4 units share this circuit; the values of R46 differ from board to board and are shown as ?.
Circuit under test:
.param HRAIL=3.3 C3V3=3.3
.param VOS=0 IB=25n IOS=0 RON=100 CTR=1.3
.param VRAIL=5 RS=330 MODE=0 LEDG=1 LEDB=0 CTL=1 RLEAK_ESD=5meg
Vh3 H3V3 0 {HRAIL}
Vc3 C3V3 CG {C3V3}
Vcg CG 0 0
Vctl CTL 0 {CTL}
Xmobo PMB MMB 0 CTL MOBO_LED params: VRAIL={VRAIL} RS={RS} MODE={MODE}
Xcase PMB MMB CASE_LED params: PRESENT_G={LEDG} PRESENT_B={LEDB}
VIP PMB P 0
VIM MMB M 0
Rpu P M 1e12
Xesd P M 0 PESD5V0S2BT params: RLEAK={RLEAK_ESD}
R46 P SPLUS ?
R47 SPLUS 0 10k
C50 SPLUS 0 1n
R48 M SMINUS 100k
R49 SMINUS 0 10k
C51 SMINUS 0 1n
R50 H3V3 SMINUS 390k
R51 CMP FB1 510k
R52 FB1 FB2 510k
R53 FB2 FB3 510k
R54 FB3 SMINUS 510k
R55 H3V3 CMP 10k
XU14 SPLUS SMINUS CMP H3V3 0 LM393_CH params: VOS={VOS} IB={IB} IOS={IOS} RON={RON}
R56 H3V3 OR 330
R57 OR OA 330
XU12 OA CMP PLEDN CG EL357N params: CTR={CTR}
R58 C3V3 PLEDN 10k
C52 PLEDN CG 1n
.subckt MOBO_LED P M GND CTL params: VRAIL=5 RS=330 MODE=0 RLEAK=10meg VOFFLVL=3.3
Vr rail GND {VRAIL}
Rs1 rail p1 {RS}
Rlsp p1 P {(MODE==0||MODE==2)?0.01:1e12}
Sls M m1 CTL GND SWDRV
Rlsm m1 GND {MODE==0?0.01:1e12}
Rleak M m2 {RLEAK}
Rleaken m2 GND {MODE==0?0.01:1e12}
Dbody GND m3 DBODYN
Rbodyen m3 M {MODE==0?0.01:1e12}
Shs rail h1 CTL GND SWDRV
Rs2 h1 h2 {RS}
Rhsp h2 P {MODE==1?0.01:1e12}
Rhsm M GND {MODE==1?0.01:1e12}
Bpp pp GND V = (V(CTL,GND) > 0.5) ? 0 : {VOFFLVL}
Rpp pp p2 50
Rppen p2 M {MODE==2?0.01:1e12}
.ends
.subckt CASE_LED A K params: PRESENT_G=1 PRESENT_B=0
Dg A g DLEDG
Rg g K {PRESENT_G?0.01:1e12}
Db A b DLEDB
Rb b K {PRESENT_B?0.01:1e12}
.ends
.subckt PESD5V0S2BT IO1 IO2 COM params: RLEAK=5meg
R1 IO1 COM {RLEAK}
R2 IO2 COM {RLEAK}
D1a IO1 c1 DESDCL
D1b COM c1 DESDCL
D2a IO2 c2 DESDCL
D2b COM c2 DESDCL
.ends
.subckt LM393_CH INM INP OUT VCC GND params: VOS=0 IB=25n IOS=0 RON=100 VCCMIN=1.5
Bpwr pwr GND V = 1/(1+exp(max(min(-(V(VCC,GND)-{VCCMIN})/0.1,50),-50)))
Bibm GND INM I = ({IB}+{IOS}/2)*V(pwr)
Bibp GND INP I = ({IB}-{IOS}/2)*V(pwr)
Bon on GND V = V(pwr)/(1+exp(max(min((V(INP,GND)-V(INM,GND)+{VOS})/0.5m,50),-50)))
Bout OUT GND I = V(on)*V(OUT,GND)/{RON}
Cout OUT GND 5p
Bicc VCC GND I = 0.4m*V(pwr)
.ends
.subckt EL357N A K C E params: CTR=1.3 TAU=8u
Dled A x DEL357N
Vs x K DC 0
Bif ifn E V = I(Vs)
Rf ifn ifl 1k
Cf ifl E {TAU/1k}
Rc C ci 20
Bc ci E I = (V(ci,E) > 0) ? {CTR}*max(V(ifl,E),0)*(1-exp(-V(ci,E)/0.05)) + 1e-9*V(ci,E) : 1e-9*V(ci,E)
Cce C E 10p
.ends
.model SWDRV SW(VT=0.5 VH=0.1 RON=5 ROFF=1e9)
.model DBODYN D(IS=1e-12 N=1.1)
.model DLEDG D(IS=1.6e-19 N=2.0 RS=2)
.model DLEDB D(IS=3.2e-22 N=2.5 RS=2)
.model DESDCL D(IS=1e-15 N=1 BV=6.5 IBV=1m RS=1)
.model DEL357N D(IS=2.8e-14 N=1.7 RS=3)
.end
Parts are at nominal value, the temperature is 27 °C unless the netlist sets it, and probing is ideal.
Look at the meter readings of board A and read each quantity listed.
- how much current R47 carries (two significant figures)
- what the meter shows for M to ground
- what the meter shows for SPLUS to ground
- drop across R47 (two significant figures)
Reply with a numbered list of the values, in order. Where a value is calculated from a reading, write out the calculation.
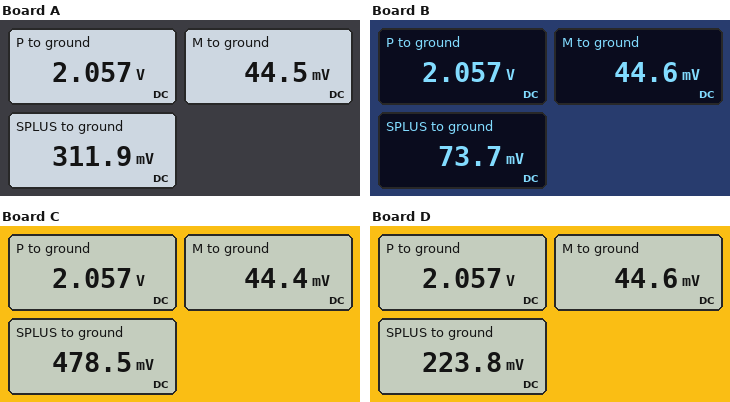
1. (311.9 mV) / 10 kΩ = 31 µA
2. 44.5 mV
3. 311.9 mV
4. 311.9 mV = 310 mV
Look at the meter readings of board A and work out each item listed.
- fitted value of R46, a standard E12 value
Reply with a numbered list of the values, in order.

1. 56 kΩ
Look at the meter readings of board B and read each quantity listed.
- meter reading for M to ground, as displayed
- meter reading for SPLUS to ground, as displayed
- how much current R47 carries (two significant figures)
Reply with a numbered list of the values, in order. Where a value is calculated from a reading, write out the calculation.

1. 44.6 mV
2. 73.7 mV
3. (73.7 mV) / 10 kΩ = 7.4 µA
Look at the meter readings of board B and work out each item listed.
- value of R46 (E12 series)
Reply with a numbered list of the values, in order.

1. 270 kΩ
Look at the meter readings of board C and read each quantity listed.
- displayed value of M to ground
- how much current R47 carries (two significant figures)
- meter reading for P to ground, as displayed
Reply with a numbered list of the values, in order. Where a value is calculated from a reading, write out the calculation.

1. 44.4 mV
2. (478.5 mV) / 10 kΩ = 48 µA
3. 2.057 V
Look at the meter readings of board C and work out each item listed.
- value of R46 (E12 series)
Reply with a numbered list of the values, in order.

1. 33 kΩ
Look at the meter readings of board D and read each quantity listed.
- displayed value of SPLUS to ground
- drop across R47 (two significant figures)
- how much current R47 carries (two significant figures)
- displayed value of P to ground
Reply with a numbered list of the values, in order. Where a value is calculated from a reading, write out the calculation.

1. 223.8 mV
2. 223.8 mV = 220 mV
3. (223.8 mV) / 10 kΩ = 22 µA
4. 2.057 V
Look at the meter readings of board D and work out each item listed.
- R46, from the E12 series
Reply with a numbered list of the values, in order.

1. 82 kΩ
